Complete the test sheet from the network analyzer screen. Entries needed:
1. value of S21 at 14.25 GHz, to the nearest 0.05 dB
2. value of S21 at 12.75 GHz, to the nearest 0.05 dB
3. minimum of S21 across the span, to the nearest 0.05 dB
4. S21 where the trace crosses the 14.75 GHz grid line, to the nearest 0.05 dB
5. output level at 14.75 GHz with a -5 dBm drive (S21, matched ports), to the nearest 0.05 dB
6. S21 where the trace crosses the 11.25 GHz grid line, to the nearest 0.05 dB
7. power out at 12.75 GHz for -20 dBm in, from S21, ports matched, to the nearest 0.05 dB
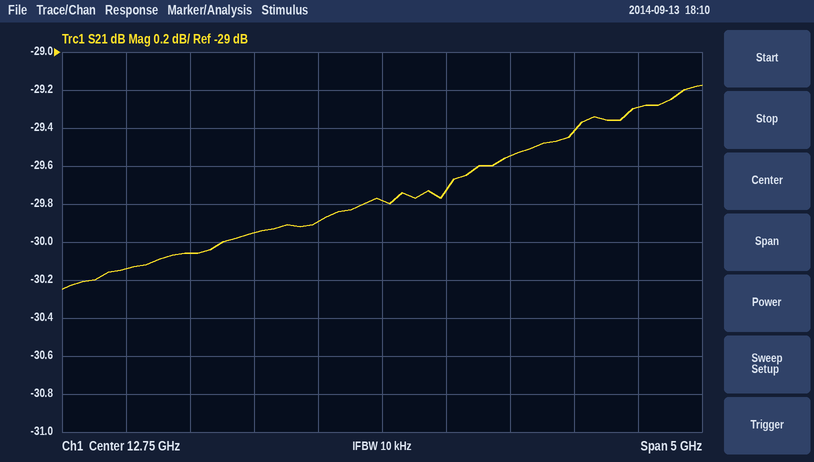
-29.40 dB
-29.80 dB
-30.25 dB
-29.30 dB
-34.30 dBm
-30.05 dB
-49.80 dBm
